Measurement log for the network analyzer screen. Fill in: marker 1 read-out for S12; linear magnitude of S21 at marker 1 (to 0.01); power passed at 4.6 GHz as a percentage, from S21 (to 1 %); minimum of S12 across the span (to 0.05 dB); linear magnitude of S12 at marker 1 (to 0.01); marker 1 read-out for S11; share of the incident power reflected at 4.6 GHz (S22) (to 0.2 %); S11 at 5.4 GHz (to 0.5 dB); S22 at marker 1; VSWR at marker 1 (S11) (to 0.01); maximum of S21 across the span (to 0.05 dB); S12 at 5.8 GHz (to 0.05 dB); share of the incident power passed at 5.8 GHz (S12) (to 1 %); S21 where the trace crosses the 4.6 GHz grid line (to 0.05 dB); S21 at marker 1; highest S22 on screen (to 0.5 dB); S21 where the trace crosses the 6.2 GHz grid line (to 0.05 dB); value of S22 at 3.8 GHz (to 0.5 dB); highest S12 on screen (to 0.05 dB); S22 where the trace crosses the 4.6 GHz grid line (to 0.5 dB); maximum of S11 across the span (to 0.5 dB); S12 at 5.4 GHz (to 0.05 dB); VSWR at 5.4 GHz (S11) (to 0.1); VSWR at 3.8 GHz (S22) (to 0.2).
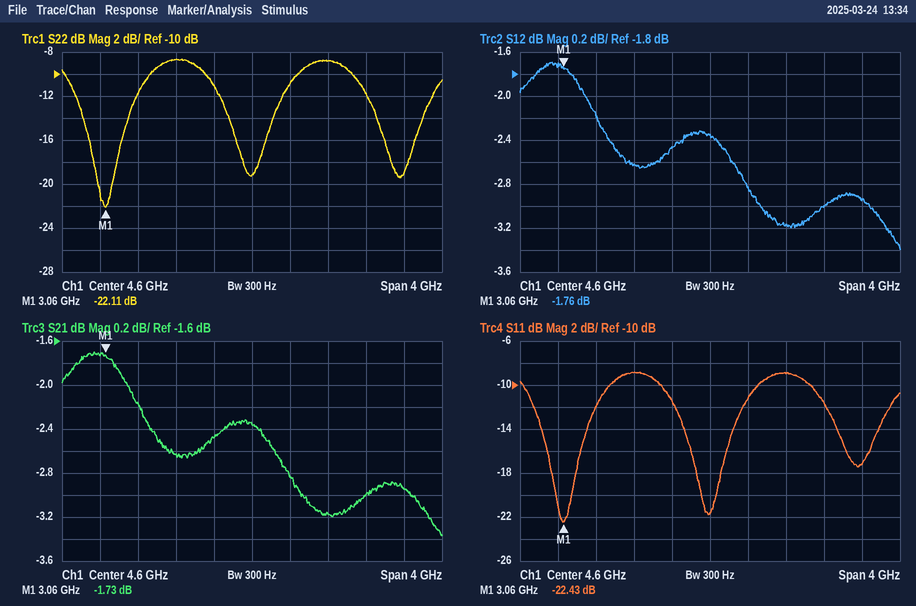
-1.76 dB
0.82
58 %
-3.40 dB
0.82
-22.43 dB
1.2 %
-9.0 dB
-22.11 dB
1.16
-1.70 dB
-3.00 dB
50 %
-2.35 dB
-1.73 dB
-8.5 dB
-2.95 dB
-8.5 dB
-1.70 dB
-19.0 dB
-9.0 dB
-3.15 dB
2.1
2.2
